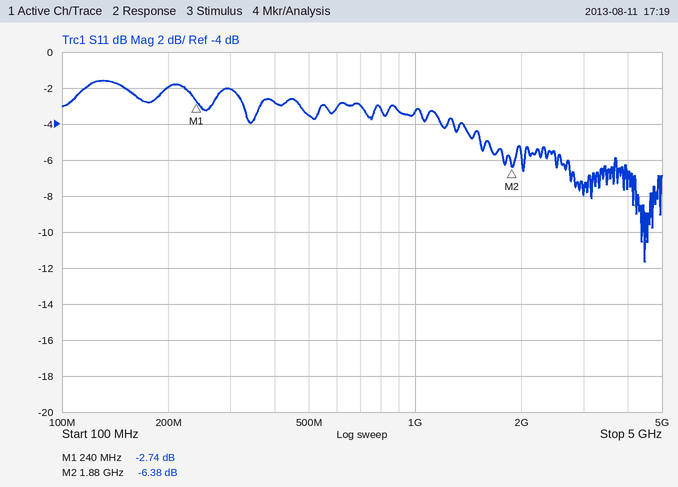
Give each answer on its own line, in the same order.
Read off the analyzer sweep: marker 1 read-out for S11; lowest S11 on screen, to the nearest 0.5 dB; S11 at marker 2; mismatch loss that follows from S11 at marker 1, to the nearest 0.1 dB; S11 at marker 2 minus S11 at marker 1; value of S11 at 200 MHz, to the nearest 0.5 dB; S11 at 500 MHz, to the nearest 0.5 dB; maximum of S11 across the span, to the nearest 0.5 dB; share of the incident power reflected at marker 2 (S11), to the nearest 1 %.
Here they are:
-2.74 dB
-11.5 dB
-6.38 dB
3.3 dB
-3.64 dB
-2.0 dB
-3.5 dB
-1.5 dB
23 %
